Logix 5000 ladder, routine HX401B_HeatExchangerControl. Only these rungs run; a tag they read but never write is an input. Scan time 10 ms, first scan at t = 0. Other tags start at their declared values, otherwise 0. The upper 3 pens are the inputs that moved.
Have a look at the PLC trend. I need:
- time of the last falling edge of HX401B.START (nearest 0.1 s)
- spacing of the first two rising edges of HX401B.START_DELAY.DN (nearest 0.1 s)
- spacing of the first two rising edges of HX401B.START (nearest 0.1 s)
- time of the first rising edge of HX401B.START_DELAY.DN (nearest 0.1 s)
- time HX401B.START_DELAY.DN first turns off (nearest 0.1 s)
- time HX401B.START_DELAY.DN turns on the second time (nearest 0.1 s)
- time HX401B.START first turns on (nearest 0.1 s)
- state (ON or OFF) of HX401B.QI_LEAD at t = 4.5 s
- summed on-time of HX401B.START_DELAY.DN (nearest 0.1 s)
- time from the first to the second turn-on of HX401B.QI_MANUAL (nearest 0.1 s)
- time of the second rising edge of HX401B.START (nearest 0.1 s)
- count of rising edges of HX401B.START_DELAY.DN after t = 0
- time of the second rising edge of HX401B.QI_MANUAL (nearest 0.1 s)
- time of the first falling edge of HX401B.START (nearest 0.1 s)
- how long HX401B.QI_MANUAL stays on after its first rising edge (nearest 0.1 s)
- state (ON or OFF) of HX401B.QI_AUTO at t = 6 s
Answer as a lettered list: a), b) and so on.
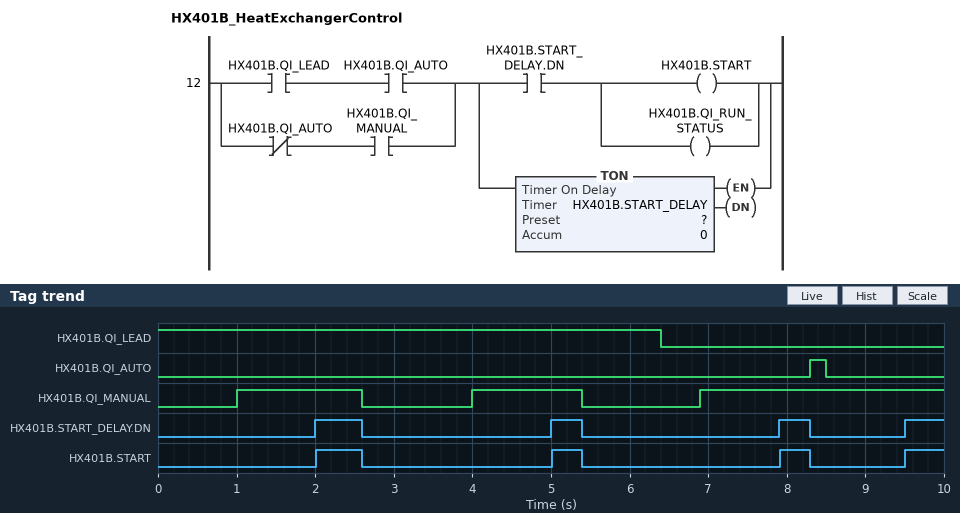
a) 8.3 s
b) 3.0 s
c) 3.0 s
d) 2.0 s
e) 2.6 s
f) 5.0 s
g) 2.0 s
h) ON
i) 1.9 s
j) 3.0 s
k) 5.0 s
l) 4
m) 4.0 s
n) 2.6 s
o) 1.6 s
p) OFF
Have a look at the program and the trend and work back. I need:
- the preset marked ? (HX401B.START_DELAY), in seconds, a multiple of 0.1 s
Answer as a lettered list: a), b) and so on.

a) 1.0 s
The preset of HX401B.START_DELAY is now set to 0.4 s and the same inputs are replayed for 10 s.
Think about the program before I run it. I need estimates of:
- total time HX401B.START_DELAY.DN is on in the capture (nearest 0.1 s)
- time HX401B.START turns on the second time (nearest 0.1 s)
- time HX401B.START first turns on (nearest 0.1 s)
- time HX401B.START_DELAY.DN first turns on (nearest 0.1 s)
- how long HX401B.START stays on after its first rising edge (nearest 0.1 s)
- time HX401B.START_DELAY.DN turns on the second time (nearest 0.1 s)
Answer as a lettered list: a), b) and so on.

a) 4.3 s
b) 4.4 s
c) 1.4 s
d) 1.4 s
e) 1.2 s
f) 4.4 s
